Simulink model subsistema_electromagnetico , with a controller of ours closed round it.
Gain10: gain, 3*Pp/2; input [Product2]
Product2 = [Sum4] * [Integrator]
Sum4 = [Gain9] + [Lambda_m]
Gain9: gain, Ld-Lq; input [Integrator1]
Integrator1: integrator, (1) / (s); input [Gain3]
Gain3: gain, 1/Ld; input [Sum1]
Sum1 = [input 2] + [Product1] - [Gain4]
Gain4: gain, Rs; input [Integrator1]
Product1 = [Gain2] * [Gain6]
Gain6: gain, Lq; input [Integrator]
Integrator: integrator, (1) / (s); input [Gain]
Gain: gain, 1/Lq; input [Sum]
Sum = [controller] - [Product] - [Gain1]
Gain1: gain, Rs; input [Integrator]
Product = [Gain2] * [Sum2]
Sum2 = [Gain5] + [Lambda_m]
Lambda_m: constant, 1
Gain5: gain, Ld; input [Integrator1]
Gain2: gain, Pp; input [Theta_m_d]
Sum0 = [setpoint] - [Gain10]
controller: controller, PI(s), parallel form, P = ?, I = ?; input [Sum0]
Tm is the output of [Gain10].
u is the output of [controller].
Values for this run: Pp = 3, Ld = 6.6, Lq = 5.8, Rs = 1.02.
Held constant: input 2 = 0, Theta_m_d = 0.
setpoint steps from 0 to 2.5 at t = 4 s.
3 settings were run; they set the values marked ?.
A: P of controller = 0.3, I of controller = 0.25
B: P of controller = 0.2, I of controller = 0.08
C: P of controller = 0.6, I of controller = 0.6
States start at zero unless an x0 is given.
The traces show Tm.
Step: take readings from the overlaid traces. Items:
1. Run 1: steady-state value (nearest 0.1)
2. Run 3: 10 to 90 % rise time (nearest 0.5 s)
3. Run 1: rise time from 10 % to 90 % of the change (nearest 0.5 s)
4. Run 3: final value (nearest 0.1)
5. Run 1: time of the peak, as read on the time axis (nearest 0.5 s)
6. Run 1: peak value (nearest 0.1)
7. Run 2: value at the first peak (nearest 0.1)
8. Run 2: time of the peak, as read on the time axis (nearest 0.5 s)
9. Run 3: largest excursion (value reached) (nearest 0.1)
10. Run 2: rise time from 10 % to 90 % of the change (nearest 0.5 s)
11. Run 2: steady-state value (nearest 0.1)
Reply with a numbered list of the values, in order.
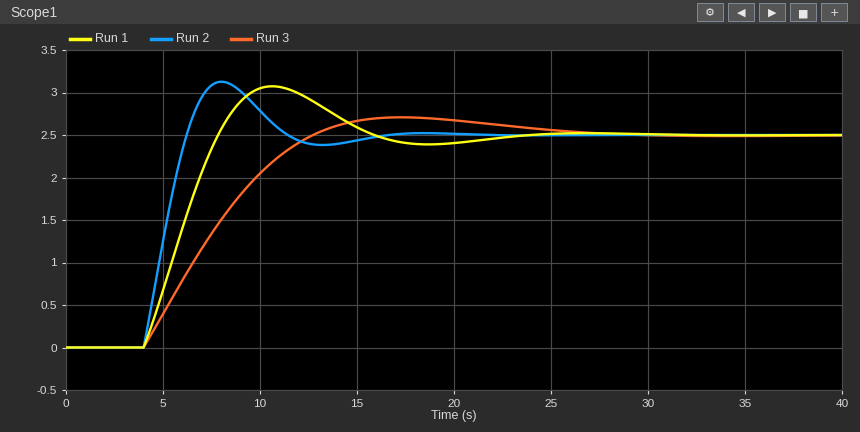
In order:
1. 2.5
2. 6.5 s
3. 3.0 s
4. 2.5
5. 10.5 s
6. 3.1
7. 3.1
8. 8.0 s
9. 2.7
10. 1.5 s
11. 2.5
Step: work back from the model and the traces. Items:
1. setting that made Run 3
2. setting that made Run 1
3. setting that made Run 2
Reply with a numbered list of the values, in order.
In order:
1. B
2. A
3. C
